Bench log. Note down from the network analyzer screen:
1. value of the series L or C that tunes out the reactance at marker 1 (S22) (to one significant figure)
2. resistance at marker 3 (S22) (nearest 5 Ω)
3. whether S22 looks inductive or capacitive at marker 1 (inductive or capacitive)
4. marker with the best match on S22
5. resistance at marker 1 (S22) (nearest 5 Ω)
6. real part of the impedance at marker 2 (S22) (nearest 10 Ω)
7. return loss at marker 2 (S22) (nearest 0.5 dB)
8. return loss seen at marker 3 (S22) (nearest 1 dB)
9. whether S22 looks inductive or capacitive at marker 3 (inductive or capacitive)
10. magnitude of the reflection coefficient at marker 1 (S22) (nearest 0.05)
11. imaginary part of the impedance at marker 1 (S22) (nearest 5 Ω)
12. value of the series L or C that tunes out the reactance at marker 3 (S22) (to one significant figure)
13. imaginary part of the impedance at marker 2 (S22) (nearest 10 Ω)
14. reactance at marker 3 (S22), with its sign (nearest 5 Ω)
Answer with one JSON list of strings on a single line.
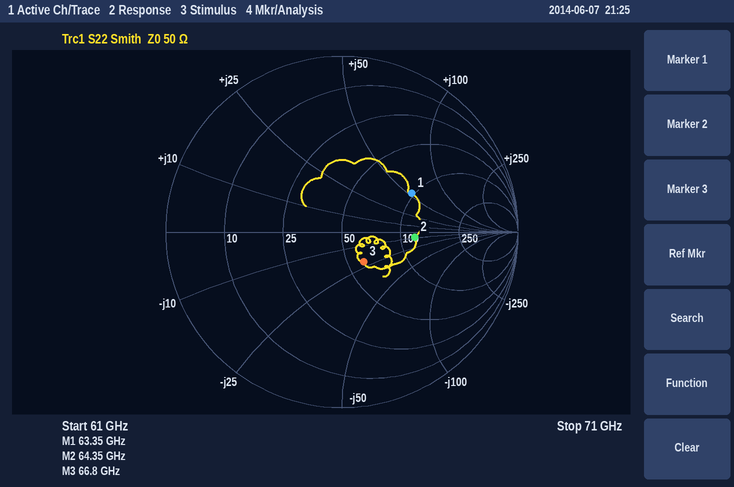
["50 fF", "60 Ω", "inductive", "marker 3", "95 Ω", "120 Ω", "7.5 dB", "14 dB", "capacitive", "0.45", "+55 Ω", "50 pH", "-10 Ω", "-20 Ω"]
